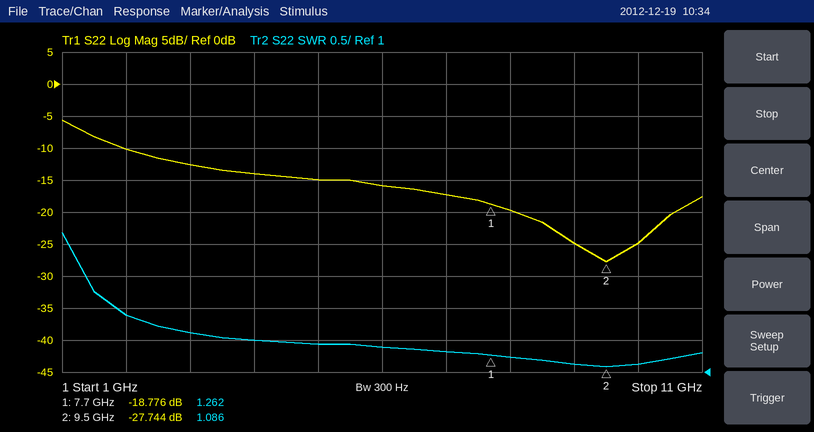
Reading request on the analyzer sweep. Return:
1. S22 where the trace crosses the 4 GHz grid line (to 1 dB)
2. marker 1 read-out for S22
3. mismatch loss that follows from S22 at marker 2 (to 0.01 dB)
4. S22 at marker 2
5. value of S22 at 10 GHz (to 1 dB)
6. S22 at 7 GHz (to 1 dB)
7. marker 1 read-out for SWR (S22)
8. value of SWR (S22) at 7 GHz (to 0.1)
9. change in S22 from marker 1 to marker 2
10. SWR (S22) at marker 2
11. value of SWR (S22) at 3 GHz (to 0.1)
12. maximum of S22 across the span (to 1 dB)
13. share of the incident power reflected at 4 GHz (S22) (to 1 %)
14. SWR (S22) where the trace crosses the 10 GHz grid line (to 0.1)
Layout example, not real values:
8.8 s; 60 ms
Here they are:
-14 dB; -18.776 dB; 0.01 dB; -27.744 dB; -25 dB; -17 dB; 1.262; 1.3; -8.968 dB; 1.086; 1.6; -6 dB; 4 %; 1.1
